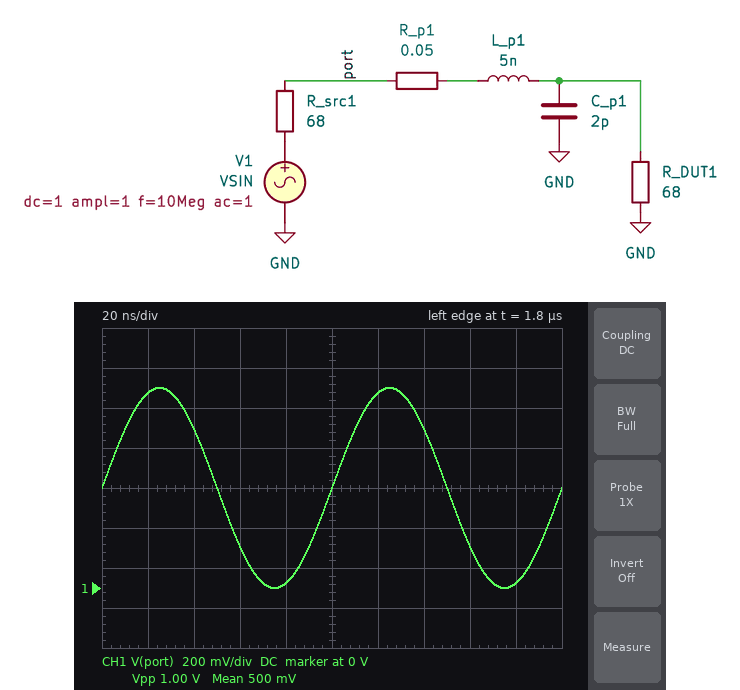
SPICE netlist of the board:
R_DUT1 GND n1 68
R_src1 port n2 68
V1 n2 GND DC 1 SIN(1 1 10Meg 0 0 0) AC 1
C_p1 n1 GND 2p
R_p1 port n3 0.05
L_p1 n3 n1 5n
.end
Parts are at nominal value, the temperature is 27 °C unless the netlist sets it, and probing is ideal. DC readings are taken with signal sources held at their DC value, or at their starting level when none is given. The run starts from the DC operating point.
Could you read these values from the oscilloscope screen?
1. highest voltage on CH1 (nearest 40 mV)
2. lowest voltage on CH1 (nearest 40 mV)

1.00 V
0 V
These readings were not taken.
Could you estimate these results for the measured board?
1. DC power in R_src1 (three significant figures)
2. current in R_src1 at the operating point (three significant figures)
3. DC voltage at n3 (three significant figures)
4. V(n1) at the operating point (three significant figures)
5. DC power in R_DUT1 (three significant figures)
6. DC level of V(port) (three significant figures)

3.67 mW
7.35 mA
500 mV
500 mV
3.67 mW
500 mV
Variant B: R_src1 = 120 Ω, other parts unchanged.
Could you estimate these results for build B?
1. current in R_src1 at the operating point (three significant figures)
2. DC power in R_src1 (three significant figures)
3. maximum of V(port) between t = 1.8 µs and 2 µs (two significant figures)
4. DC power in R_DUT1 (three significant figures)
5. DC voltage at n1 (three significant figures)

5.32 mA
3.39 mW
720 mV
1.92 mW
362 mV
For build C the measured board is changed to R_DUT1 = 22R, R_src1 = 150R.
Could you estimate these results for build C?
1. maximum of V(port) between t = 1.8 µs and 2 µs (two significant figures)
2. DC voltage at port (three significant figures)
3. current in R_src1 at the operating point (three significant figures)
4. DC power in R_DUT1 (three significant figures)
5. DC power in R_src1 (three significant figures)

260 mV
128 mV
5.81 mA
743 µW
5.07 mW
